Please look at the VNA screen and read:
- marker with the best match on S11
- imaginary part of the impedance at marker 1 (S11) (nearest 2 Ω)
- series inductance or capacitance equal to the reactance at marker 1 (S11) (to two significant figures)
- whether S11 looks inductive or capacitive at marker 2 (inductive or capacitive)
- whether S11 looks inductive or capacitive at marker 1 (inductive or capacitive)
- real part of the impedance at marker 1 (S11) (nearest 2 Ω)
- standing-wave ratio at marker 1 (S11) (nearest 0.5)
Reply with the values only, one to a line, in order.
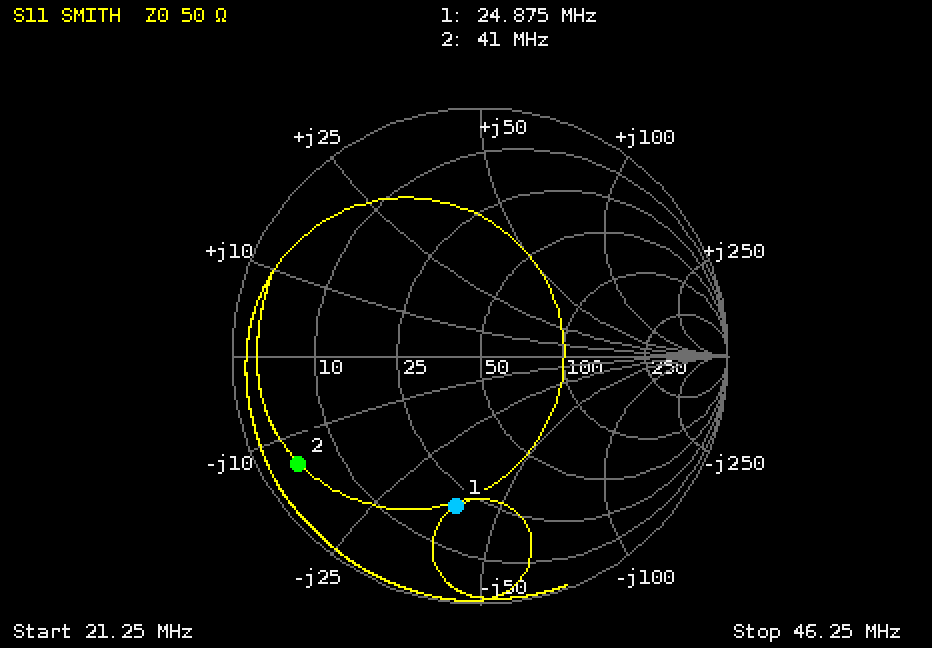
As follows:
marker 1
-38 Ω
170 pF
capacitive
capacitive
20 Ω
4.0
